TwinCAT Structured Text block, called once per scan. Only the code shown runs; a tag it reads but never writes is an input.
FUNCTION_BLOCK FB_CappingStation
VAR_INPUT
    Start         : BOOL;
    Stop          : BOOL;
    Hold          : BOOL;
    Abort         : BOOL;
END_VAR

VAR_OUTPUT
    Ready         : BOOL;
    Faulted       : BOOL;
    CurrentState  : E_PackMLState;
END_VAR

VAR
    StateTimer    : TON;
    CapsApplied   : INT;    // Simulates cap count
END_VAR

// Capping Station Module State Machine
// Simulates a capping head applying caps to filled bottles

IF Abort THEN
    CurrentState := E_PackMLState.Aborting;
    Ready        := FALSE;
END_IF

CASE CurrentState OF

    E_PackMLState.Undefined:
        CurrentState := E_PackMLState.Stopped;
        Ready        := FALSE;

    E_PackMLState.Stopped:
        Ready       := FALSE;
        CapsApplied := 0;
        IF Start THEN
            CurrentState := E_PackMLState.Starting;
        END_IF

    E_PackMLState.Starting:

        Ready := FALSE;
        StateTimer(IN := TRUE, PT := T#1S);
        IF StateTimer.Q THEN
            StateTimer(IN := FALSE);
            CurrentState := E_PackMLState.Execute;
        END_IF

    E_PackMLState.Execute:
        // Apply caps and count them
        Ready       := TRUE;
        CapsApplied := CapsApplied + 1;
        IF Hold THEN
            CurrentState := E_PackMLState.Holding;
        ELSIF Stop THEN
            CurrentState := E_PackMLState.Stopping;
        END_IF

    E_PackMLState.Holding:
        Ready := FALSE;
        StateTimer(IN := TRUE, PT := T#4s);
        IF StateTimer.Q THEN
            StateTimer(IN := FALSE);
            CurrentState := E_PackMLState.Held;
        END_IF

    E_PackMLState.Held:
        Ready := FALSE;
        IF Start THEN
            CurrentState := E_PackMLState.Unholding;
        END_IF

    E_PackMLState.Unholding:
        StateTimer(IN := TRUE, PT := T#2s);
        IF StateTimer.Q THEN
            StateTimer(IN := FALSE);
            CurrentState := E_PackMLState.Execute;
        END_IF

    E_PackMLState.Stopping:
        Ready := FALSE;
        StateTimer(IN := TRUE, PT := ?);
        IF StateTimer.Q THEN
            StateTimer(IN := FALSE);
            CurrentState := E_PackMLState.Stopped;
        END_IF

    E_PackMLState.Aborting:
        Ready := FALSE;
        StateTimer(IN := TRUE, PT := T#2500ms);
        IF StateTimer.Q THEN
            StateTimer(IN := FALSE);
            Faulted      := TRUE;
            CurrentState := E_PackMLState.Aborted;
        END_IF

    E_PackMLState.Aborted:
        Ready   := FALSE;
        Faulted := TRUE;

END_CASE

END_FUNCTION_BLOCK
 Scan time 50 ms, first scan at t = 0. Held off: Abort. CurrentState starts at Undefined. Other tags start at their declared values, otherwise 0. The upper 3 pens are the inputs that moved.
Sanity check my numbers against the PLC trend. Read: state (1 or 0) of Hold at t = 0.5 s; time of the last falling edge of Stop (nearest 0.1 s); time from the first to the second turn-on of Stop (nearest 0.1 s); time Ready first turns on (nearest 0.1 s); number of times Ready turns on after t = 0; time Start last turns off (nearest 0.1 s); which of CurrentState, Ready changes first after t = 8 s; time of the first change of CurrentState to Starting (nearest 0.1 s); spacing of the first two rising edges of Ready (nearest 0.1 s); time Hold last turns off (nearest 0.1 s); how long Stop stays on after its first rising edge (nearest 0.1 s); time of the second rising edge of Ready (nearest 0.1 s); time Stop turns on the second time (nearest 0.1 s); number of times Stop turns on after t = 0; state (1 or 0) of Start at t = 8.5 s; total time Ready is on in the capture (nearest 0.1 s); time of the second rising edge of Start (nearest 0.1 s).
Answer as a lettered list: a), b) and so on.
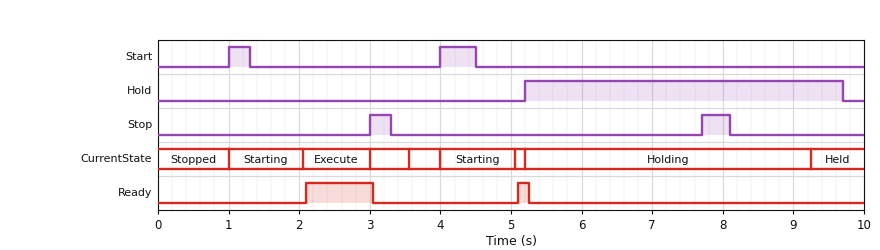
a) 0
b) 8.1 s
c) 4.7 s
d) 2.1 s
e) 2
f) 4.5 s
g) CurrentState
h) 1.0 s
i) 3.0 s
j) 9.7 s
k) 0.3 s
l) 5.1 s
m) 7.7 s
n) 2
o) 0
p) 1.1 s
q) 4.0 s
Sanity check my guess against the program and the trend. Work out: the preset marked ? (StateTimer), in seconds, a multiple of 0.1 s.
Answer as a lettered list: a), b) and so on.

a) 0.5 s
